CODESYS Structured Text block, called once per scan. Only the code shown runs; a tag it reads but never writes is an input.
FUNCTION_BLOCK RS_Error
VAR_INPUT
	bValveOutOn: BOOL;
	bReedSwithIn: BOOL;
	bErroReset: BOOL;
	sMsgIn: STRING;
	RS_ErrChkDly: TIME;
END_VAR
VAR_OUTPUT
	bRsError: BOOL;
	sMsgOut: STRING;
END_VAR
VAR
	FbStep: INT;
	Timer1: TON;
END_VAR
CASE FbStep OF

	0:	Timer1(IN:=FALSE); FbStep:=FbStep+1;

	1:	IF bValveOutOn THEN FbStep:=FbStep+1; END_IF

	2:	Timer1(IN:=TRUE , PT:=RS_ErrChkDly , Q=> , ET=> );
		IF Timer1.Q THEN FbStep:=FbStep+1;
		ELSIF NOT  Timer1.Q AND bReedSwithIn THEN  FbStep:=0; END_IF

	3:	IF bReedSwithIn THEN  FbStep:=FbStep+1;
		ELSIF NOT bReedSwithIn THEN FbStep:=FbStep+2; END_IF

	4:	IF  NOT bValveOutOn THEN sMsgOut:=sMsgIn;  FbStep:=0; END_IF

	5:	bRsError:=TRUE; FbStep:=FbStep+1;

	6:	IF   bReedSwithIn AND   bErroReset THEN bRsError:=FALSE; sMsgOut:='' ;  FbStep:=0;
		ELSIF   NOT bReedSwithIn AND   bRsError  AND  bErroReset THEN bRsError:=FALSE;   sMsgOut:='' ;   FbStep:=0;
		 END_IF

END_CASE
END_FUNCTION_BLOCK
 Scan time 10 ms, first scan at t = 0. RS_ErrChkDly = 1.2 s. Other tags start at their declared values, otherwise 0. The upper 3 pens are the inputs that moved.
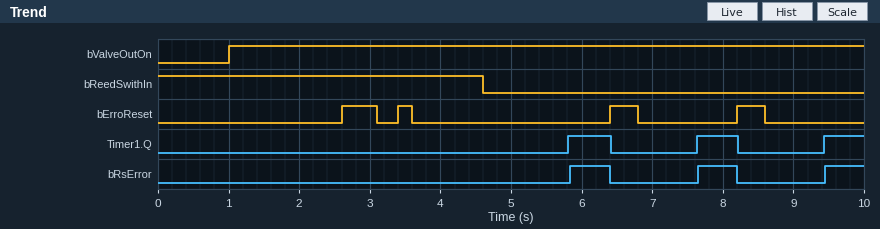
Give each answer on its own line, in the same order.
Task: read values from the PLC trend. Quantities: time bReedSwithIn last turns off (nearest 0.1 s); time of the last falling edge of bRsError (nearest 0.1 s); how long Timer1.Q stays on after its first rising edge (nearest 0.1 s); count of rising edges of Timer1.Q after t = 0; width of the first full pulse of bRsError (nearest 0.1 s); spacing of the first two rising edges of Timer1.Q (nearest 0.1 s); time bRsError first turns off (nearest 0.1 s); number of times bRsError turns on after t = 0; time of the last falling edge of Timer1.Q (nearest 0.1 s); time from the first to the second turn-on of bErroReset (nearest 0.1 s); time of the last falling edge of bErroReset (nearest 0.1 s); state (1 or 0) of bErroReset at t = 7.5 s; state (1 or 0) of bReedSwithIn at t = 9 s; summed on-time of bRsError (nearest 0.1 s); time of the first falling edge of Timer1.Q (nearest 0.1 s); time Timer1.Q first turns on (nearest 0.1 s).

4.6 s
8.2 s
0.6 s
3
0.6 s
1.8 s
6.4 s
3
8.2 s
0.8 s
8.6 s
0
0
1.7 s
6.4 s
5.8 s
